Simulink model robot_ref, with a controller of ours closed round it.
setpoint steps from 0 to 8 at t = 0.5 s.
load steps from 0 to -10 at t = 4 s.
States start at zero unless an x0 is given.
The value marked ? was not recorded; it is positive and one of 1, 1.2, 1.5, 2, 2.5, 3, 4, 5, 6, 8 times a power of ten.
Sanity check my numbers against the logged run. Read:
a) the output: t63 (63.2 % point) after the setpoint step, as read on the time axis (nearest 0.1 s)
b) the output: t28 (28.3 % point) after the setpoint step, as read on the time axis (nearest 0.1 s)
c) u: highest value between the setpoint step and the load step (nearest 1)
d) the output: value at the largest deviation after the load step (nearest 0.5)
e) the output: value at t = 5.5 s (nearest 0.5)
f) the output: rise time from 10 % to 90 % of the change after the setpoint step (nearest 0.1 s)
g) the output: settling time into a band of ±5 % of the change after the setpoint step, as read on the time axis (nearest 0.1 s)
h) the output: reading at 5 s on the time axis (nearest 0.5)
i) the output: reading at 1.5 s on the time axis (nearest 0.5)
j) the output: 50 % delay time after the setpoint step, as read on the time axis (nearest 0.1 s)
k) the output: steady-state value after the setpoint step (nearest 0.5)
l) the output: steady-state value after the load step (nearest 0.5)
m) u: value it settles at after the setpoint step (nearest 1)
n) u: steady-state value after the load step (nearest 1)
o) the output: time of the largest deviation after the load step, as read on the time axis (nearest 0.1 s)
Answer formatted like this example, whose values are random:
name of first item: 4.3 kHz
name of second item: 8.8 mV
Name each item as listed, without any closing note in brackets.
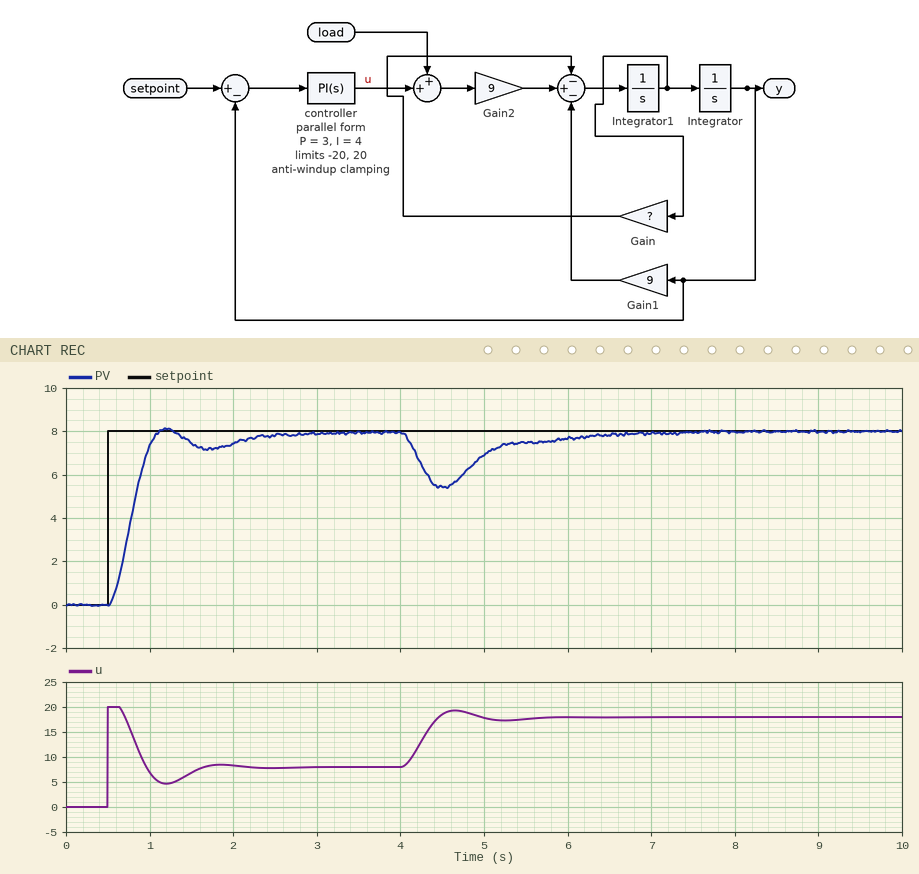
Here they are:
the output: t63 (63.2 % point) after the setpoint step, as read on the time axis: 0.8 s
the output: t28 (28.3 % point) after the setpoint step, as read on the time axis: 0.7 s
u: highest value between the setpoint step and the load step: 20
the output: value at the largest deviation after the load step: 5.5
the output: value at t = 5.5 s: 7.5
the output: rise time from 10 % to 90 % of the change after the setpoint step: 0.4 s
the output: settling time into a band of ±5 % of the change after the setpoint step, as read on the time axis: 2.1 s
the output: reading at 5 s on the time axis: 7.0
the output: reading at 1.5 s on the time axis: 7.5
the output: 50 % delay time after the setpoint step, as read on the time axis: 0.8 s
the output: steady-state value after the setpoint step: 8.0
the output: steady-state value after the load step: 8.0
u: value it settles at after the setpoint step: 8
u: steady-state value after the load step: 18
the output: time of the largest deviation after the load step, as read on the time axis: 4.5 s
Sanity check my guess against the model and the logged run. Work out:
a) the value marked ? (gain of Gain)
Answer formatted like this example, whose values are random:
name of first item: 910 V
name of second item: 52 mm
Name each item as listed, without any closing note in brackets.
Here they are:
the value marked ?: 6
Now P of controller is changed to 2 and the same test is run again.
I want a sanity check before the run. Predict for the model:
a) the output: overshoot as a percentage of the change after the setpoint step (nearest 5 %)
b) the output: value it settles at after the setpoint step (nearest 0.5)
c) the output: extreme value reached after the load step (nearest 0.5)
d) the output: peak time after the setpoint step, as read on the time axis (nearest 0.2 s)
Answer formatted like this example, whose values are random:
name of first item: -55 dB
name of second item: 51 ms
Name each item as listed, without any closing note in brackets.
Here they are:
the output: overshoot as a percentage of the change after the setpoint step: 15 %
the output: value it settles at after the setpoint step: 8.0
the output: extreme value reached after the load step: 5.0
the output: peak time after the setpoint step, as read on the time axis: 1.4 s
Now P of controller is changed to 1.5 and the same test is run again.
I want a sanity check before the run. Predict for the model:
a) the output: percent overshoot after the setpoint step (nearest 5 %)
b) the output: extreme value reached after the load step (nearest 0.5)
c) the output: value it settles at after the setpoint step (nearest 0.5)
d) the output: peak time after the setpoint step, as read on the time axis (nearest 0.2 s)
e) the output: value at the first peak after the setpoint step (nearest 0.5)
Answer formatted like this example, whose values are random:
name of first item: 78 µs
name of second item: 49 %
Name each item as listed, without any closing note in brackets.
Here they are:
the output: percent overshoot after the setpoint step: 20 %
the output: extreme value reached after the load step: 4.5
the output: value it settles at after the setpoint step: 8.0
the output: peak time after the setpoint step, as read on the time axis: 1.4 s
the output: value at the first peak after the setpoint step: 9.5
